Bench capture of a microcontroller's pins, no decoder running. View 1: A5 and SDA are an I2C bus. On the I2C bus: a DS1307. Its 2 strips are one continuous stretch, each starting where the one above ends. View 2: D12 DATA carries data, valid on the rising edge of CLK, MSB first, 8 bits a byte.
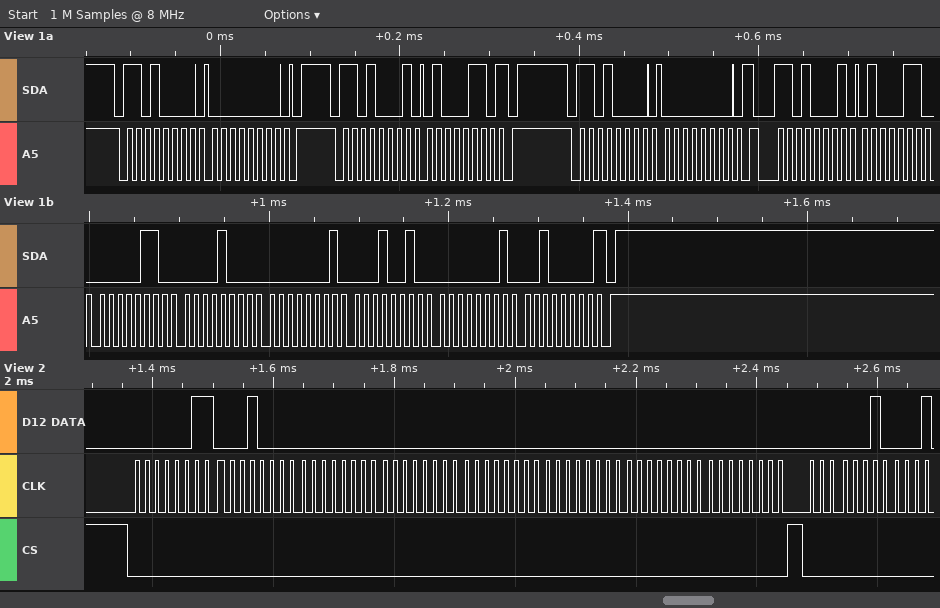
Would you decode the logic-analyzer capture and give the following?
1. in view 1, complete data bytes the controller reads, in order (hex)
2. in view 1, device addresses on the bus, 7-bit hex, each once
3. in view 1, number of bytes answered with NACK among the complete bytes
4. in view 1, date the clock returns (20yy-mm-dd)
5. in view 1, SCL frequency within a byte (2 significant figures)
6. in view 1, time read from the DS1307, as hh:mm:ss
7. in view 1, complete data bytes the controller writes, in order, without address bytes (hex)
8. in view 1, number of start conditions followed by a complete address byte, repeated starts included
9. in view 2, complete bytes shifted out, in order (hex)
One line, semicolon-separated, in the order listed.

46 46 06 08 01 12 01 20; 0x68; 2; 2020-01-12; 100 kHz; 08:06:46; 00 00; 4; 03 10 00 00 00 00 00 00 02
